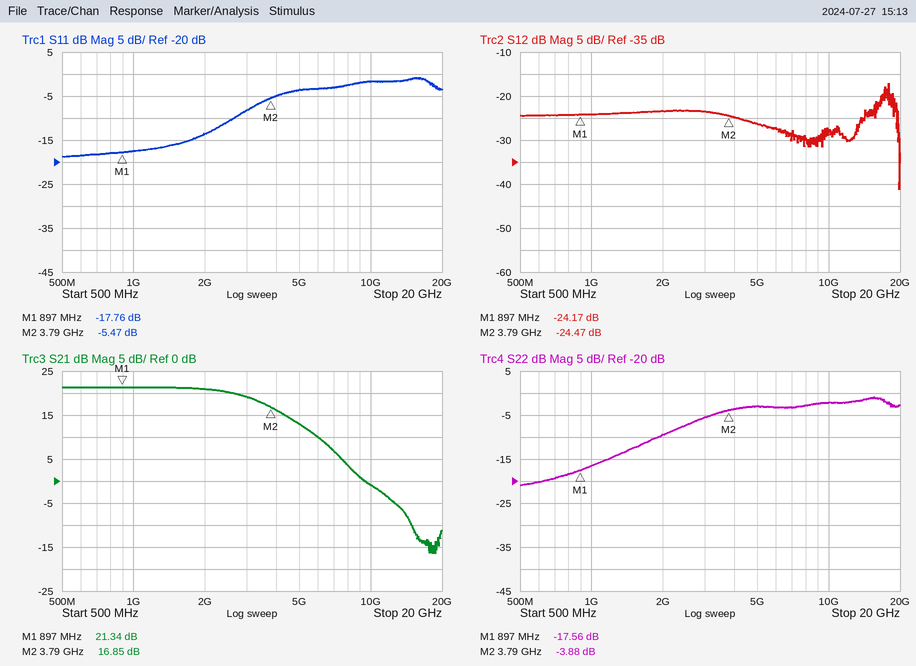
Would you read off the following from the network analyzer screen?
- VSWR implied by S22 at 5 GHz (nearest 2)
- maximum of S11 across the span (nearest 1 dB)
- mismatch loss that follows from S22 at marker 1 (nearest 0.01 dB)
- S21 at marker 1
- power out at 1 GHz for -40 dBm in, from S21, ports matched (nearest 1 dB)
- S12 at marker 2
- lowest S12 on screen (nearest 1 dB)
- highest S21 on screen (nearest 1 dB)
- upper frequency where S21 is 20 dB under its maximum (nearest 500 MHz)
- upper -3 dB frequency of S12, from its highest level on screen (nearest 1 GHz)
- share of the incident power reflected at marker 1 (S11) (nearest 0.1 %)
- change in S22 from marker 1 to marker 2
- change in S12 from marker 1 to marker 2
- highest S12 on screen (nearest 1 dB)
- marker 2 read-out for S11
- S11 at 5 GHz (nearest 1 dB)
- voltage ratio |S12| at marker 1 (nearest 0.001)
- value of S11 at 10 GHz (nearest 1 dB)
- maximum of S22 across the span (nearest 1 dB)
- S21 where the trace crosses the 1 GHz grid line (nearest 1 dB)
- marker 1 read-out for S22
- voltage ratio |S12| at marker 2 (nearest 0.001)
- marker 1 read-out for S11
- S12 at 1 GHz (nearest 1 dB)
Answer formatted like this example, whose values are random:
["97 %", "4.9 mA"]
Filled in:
["6", "-1 dB", "0.08 dB", "21.34 dB", "-19 dBm", "-24.47 dB", "-41 dB", "21 dB", "9.0 GHz", "18 GHz", "1.7 %", "13.68 dB", "-0.30 dB", "-17 dB", "-5.47 dB", "-4 dB", "0.062", "-2 dB", "-1 dB", "21 dB", "-17.56 dB", "0.060", "-17.76 dB", "-24 dB"]
